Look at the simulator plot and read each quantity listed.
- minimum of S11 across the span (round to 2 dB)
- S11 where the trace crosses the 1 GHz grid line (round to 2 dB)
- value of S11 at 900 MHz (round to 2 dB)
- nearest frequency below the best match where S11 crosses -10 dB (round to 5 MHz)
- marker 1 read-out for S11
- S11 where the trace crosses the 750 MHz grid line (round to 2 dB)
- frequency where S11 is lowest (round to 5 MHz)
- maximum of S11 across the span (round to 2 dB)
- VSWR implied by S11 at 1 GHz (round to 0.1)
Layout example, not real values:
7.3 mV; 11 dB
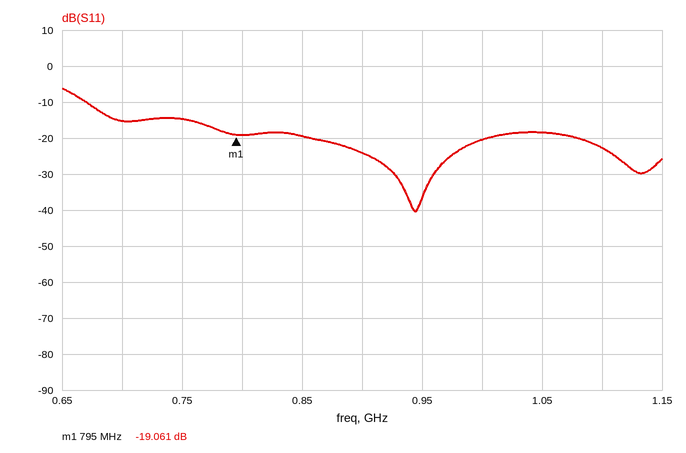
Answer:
-40 dB; -20 dB; -24 dB; 670 MHz; -19.061 dB; -14 dB; 945 MHz; -6 dB; 1.2
